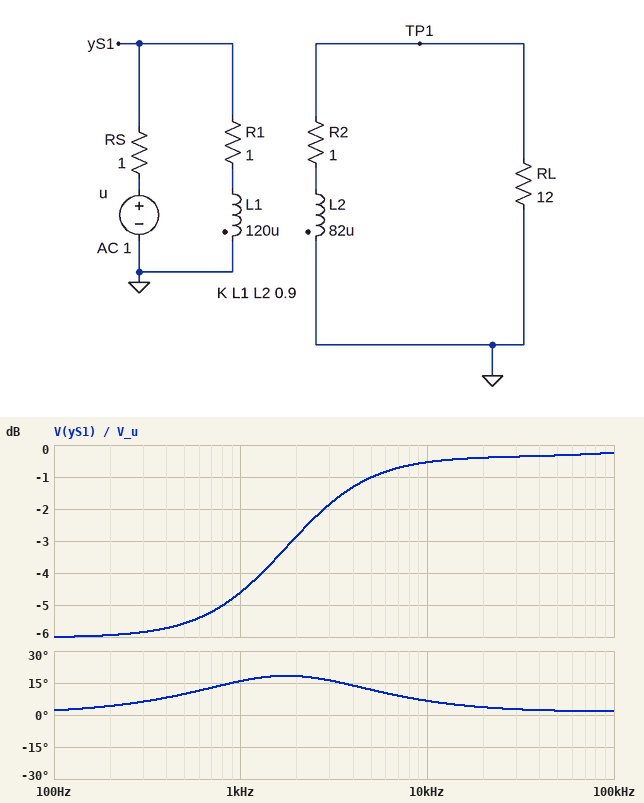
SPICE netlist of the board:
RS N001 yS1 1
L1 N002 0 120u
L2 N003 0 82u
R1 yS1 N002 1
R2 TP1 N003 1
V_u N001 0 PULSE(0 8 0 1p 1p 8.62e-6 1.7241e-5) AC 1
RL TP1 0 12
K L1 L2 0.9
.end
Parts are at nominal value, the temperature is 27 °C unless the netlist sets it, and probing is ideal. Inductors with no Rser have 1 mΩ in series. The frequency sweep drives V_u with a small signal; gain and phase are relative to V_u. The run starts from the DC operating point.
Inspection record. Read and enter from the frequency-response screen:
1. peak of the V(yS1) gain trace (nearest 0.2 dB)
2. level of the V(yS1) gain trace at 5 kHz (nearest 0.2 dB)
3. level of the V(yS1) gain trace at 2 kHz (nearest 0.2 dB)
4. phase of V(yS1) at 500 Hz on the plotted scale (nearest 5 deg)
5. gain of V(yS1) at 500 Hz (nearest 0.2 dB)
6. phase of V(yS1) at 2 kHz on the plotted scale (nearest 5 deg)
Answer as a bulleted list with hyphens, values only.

- -0.2 dB
- -1.0 dB
- -2.8 dB
- 10 deg
- -5.6 dB
- 20 deg
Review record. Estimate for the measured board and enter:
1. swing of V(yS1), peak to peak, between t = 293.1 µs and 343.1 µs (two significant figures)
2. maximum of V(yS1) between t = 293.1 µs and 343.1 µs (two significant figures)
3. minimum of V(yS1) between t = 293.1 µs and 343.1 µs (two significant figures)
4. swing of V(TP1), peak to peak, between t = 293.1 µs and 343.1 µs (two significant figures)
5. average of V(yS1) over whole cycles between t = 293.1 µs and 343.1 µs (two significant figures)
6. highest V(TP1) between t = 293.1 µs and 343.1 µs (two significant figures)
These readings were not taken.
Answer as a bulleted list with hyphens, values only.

- 8.6 V
- 6.3 V
- -2.3 V
- 5.0 V
- 2.0 V
- 2.5 V
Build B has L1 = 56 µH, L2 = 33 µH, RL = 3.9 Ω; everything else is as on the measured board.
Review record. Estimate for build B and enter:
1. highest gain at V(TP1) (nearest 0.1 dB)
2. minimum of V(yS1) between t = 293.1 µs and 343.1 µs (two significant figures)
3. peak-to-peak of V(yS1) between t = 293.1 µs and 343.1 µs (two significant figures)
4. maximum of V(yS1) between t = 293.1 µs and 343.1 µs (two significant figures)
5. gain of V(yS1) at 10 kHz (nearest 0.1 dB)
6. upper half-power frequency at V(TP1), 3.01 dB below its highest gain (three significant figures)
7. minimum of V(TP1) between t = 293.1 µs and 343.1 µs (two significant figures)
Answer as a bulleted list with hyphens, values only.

- -7.1 dB
- -2.6 V
- 9.1 V
- 6.6 V
- -1.4 dB
- 159 kHz
- -1.8 V
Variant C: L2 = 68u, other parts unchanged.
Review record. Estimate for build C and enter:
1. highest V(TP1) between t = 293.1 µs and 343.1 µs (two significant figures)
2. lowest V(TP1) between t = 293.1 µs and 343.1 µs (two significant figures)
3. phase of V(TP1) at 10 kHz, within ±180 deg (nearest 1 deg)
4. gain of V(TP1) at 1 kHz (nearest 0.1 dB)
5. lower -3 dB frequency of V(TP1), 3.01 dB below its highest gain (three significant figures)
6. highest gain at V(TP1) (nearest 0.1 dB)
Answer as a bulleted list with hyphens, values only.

- 2.3 V
- -2.3 V
- 11 deg
- -13.2 dB
- 2.41 kHz
- -4.8 dB
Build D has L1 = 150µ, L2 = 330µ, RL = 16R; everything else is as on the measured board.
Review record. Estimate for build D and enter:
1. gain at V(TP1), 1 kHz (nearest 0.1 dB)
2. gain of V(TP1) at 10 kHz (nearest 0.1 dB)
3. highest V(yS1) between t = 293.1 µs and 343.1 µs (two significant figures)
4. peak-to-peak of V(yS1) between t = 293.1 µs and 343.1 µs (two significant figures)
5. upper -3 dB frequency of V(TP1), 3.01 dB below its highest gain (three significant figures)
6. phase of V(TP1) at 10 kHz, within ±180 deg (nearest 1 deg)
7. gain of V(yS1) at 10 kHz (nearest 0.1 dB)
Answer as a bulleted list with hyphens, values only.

- -5.8 dB
- 0 dB
- 6.5 V
- 8.8 V
- 56.0 kHz
- -1 deg
- -0.9 dB
